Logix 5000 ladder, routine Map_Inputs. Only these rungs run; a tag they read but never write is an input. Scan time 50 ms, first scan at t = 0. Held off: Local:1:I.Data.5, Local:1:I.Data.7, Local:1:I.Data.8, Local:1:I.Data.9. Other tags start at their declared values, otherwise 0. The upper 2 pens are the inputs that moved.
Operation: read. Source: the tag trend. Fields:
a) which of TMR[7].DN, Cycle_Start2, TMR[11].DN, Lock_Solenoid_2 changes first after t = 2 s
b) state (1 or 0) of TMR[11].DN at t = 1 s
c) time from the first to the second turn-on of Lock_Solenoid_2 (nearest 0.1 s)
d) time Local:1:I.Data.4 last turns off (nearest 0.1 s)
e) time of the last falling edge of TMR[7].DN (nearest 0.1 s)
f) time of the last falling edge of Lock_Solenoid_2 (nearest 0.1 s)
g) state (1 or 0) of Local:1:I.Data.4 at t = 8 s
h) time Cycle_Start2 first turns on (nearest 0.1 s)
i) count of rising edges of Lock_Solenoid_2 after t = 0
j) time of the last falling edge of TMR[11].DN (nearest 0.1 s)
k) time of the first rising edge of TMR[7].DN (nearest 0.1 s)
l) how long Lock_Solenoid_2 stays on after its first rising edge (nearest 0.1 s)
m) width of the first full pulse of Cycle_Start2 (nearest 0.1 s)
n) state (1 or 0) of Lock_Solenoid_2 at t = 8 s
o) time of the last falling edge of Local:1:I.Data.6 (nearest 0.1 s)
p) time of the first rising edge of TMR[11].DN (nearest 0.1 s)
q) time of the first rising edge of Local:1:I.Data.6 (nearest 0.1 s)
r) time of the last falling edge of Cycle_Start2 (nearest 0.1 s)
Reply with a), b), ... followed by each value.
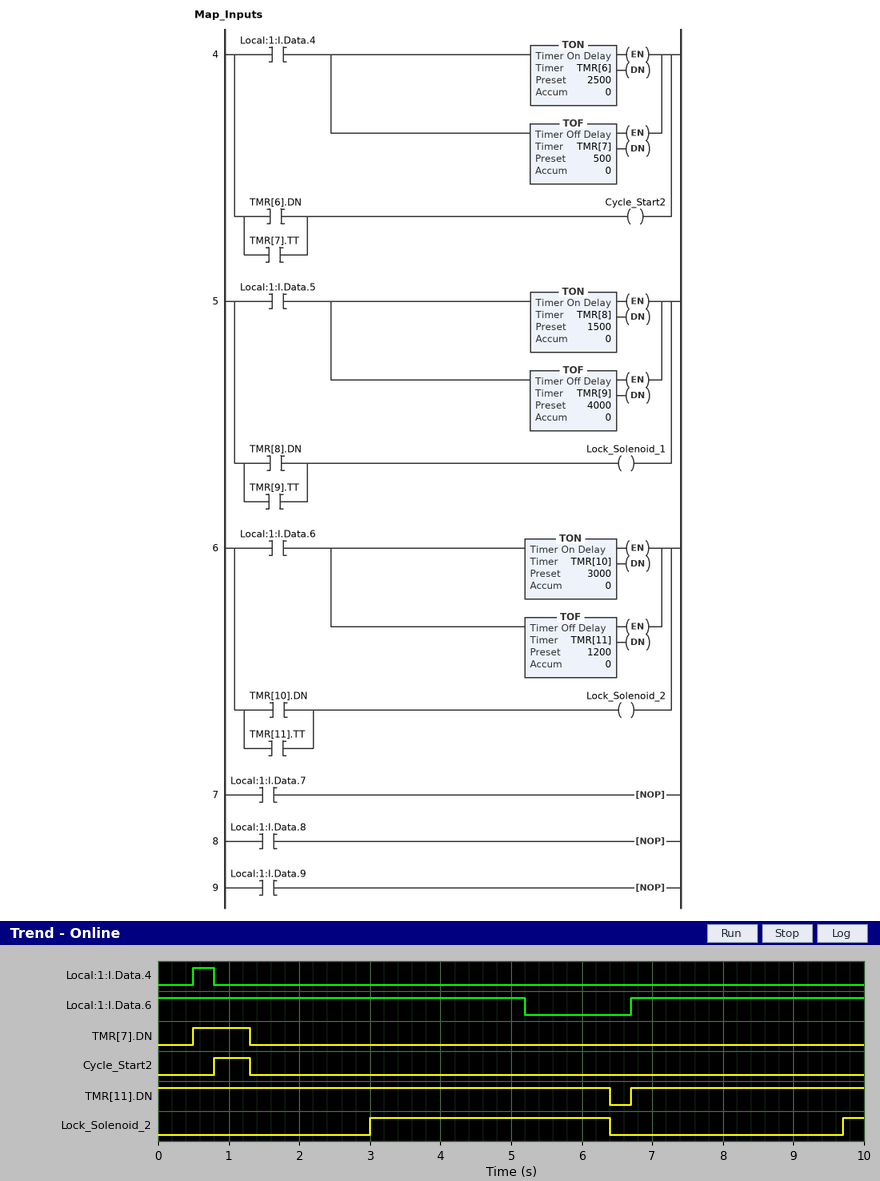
a) Lock_Solenoid_2
b) 1
c) 6.7 s
d) 0.8 s
e) 1.3 s
f) 6.4 s
g) 0
h) 0.8 s
i) 2
j) 6.4 s
k) 0.5 s
l) 3.4 s
m) 0.5 s
n) 0
o) 5.2 s
p) 6.7 s
q) 6.7 s
r) 1.3 s
